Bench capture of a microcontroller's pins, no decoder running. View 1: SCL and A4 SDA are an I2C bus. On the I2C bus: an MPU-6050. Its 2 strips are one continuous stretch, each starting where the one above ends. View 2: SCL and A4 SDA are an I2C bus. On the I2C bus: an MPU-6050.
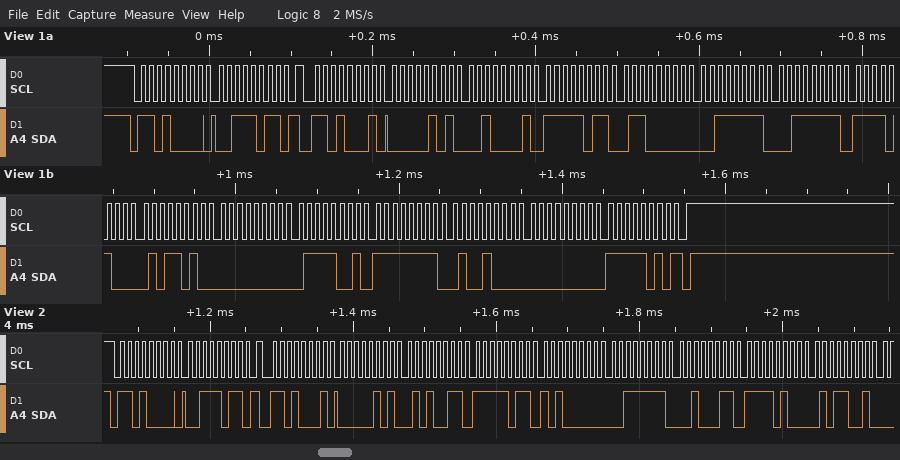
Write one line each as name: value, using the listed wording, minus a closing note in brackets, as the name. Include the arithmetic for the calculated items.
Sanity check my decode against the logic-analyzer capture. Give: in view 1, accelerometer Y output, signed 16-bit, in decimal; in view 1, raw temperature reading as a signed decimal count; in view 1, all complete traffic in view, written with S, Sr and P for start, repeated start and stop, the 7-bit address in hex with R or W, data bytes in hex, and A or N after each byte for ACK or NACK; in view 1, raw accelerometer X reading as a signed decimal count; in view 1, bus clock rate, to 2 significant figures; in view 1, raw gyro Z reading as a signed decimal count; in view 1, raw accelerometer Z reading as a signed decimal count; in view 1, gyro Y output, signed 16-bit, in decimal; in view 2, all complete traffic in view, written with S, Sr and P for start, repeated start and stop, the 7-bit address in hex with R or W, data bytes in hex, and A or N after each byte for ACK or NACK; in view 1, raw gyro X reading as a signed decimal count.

in view 1, accelerometer Y output, signed 16-bit, in decimal: 0xFB60 = -1184
in view 1, raw temperature reading as a signed decimal count: 0xF45A = -2982
in view 1, all complete traffic in view, written with S, Sr and P for start, repeated start and stop, the 7-bit address in hex with R or W, data bytes in hex, and A or N after each byte for ACK or NACK: S 68W A 3B A Sr 68R A 05 A 21 A FB A 60 A 3F A 3F A F4 A 5A A 00 A 79 A FF A 48 A 00 A FA N P
in view 1, raw accelerometer X reading as a signed decimal count: 0x0521 = 1313
in view 1, bus clock rate, to 2 significant figures: 100 kHz
in view 1, raw gyro Z reading as a signed decimal count: 0x00FA = 250
in view 1, raw accelerometer Z reading as a signed decimal count: 0x3F3F = 16191
in view 1, gyro Y output, signed 16-bit, in decimal: 0xFF48 = -184
in view 2, all complete traffic in view, written with S, Sr and P for start, repeated start and stop, the 7-bit address in hex with R or W, data bytes in hex, and A or N after each byte for ACK or NACK: S 68W A 3B A Sr 68R A 05 A 53 A FB A A0 A 3F A 23 A F4 A 59 A
in view 1, raw gyro X reading as a signed decimal count: 0x0079 = 121
